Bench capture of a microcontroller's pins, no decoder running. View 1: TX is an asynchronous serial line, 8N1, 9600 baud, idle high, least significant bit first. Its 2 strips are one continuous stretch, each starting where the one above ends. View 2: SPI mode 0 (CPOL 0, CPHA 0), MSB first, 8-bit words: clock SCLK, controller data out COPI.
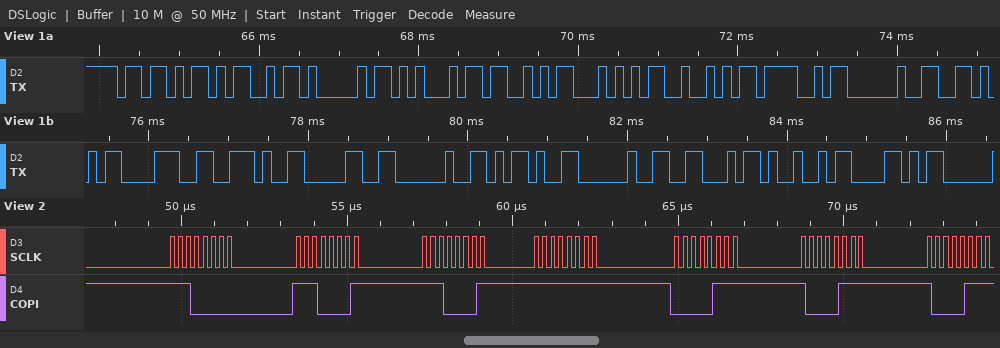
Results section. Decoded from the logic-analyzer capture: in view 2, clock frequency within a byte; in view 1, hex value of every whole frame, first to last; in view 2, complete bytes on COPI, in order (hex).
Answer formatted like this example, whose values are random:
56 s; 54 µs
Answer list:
4 MHz; 5B 4D 41 45 53 54 52 4F 20 56 38 2E 30 20 2D 20 46 49 58; E0 E1 E1 FF 07 87 87
